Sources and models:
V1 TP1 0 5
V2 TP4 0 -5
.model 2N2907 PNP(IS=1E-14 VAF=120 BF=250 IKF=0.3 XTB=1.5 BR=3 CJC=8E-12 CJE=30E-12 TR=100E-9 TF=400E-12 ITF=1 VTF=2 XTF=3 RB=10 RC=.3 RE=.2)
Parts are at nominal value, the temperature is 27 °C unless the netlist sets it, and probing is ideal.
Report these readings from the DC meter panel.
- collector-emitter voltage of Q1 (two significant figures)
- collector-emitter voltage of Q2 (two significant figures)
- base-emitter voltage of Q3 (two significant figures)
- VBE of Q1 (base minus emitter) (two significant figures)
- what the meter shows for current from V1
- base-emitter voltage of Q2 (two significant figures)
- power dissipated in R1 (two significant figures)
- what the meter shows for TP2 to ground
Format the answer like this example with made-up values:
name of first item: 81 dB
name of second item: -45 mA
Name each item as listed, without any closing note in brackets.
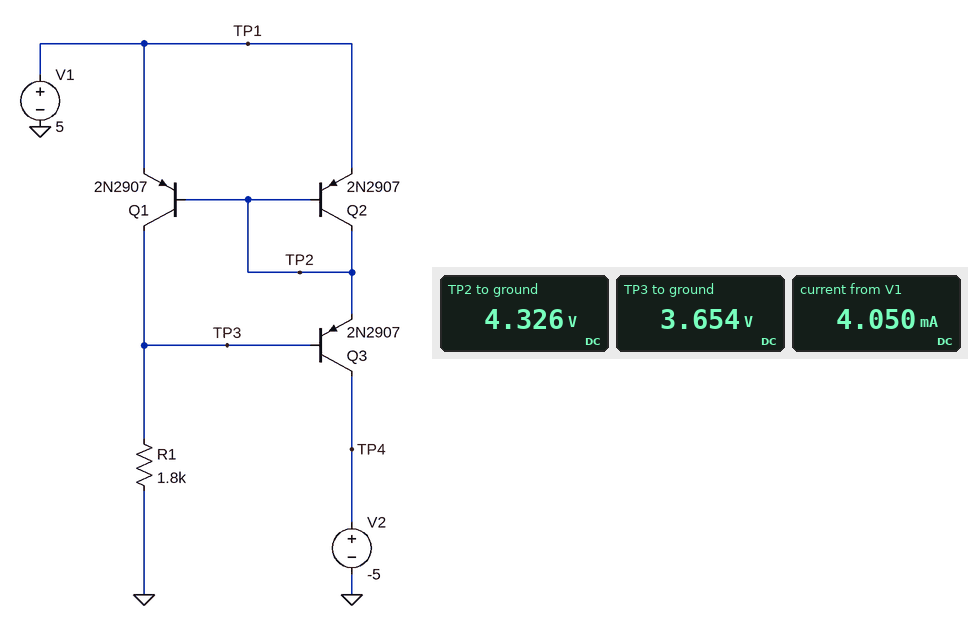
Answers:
collector-emitter voltage of Q1: -1.3 V
collector-emitter voltage of Q2: -670 mV
base-emitter voltage of Q3: -670 mV
VBE of Q1 (base minus emitter): -670 mV
what the meter shows for current from V1: 4.050 mA
base-emitter voltage of Q2: -670 mV
power dissipated in R1: 7.4 mW
what the meter shows for TP2 to ground: 4.326 V
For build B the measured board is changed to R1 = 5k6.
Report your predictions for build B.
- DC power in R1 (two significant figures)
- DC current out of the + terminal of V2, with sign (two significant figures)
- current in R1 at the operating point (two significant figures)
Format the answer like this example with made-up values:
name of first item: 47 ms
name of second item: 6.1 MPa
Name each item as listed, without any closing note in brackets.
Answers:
DC power in R1: 2.5 mW
DC current out of the + terminal of V2, with sign: -660 µA
current in R1 at the operating point: 660 µA
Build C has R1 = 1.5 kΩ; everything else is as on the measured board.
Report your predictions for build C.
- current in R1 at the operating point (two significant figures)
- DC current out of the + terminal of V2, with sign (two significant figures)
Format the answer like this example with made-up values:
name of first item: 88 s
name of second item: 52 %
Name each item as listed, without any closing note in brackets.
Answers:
current in R1 at the operating point: 2.4 mA
DC current out of the + terminal of V2, with sign: -2.4 mA
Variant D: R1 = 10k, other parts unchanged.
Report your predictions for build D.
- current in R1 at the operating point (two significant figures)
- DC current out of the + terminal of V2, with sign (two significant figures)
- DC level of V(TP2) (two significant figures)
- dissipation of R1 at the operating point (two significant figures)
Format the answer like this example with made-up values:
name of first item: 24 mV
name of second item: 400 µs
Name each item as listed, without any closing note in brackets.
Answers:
current in R1 at the operating point: 370 µA
DC current out of the + terminal of V2, with sign: -370 µA
DC level of V(TP2): 4.4 V
dissipation of R1 at the operating point: 1.4 mW
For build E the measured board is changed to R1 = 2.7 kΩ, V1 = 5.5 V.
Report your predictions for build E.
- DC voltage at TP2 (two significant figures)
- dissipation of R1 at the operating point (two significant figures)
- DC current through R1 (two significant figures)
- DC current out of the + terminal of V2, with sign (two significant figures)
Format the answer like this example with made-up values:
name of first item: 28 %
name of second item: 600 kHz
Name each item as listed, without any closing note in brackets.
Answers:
DC voltage at TP2: 4.8 V
dissipation of R1 at the operating point: 6.4 mW
DC current through R1: 1.5 mA
DC current out of the + terminal of V2, with sign: -1.5 mA
